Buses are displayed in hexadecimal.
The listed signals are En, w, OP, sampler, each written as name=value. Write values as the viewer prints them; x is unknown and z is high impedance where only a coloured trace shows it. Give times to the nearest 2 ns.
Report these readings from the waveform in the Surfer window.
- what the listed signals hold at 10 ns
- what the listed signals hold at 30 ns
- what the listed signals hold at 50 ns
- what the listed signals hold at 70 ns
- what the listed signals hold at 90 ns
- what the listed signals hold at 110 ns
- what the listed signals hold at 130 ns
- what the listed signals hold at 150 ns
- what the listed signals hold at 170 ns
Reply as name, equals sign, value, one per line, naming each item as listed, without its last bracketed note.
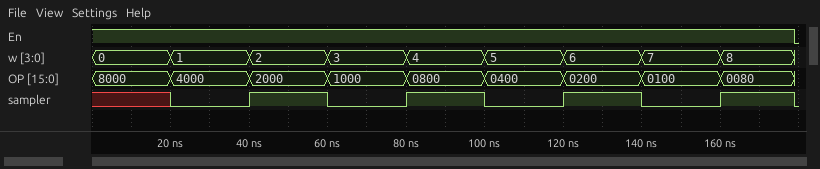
what the listed signals hold at 10 ns = En=1, w=0, OP=8000, sampler=x
what the listed signals hold at 30 ns = En=1, w=1, OP=4000, sampler=0
what the listed signals hold at 50 ns = En=1, w=2, OP=2000, sampler=1
what the listed signals hold at 70 ns = En=1, w=3, OP=1000, sampler=0
what the listed signals hold at 90 ns = En=1, w=4, OP=0800, sampler=1
what the listed signals hold at 110 ns = En=1, w=5, OP=0400, sampler=0
what the listed signals hold at 130 ns = En=1, w=6, OP=0200, sampler=1
what the listed signals hold at 150 ns = En=1, w=7, OP=0100, sampler=0
what the listed signals hold at 170 ns = En=1, w=8, OP=0080, sampler=1
